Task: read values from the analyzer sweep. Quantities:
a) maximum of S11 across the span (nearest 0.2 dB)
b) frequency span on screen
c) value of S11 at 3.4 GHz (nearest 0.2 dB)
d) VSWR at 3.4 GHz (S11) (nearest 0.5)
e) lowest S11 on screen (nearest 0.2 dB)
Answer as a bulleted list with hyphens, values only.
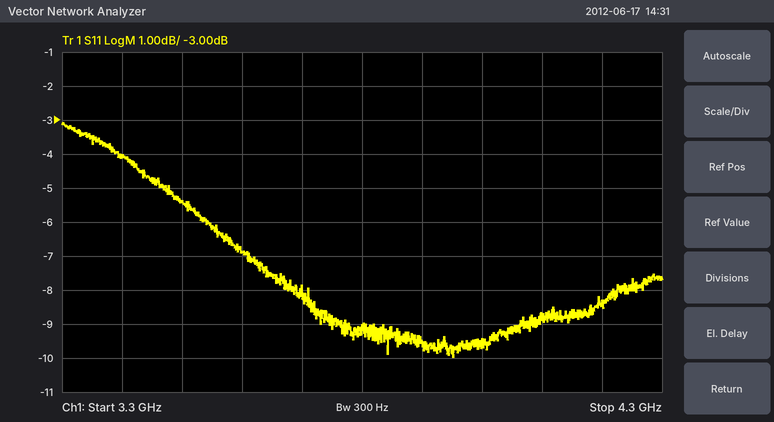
- -3.0 dB
- 1 GHz
- -4.0 dB
- 4.5
- -10.0 dB
